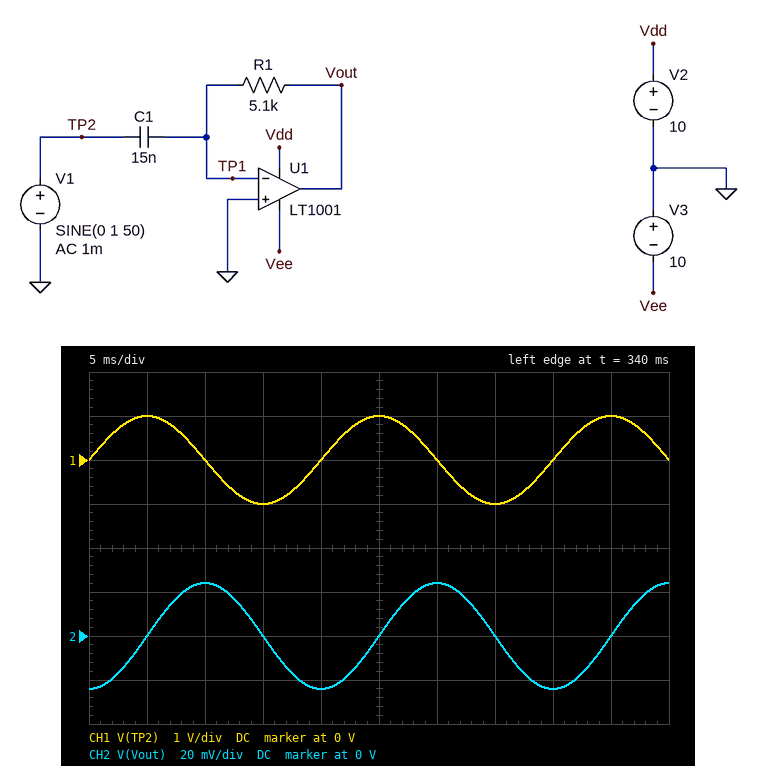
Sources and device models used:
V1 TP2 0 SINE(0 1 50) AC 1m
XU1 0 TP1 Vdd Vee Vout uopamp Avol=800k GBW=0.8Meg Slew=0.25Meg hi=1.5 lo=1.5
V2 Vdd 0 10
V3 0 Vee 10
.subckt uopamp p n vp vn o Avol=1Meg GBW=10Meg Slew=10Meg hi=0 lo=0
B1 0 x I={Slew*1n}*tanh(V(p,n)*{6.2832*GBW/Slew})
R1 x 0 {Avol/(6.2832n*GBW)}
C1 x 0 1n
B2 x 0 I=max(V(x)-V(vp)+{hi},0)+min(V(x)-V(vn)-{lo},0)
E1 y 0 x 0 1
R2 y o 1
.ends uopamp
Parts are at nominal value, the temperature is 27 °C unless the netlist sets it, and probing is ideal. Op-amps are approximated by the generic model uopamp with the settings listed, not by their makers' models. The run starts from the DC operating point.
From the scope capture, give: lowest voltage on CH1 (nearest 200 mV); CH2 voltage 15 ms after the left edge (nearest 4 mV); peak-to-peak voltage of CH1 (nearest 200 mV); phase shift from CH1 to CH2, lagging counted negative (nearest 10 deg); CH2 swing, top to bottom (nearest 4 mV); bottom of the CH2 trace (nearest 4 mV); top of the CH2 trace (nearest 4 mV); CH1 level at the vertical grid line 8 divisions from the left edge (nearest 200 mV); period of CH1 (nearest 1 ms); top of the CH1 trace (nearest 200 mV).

-1.0 V
0 V
2.0 V
-90 deg
48 mV
-24 mV
24 mV
0 V
20 ms
1.0 V
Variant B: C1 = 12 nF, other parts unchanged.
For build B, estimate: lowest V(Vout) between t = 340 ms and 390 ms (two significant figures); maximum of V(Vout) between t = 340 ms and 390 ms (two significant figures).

-19 mV
19 mV
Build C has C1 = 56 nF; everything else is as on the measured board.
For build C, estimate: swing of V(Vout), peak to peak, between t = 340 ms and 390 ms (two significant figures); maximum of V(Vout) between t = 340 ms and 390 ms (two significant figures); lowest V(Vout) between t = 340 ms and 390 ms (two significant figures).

180 mV
90 mV
-90 mV
